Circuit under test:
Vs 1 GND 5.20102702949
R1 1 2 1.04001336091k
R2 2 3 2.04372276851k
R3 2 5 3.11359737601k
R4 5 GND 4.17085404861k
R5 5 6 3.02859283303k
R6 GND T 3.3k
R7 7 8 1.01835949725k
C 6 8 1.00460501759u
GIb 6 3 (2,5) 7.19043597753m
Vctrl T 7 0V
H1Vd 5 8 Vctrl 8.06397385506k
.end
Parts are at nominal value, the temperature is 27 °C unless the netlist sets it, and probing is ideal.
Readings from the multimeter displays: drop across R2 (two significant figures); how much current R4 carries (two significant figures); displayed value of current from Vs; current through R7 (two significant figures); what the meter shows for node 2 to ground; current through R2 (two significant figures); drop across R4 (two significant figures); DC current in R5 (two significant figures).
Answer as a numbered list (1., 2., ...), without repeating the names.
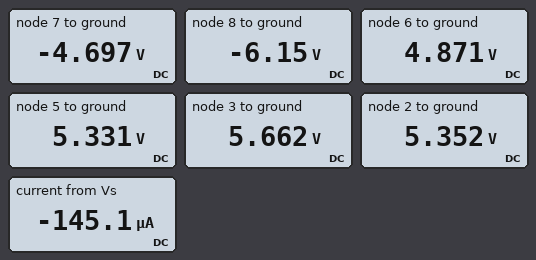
1. 310 mV
2. 1.3 mA
3. -145.1 µA
4. 1.4 mA
5. 5.352 V
6. 150 µA
7. 5.3 V
8. 150 µA
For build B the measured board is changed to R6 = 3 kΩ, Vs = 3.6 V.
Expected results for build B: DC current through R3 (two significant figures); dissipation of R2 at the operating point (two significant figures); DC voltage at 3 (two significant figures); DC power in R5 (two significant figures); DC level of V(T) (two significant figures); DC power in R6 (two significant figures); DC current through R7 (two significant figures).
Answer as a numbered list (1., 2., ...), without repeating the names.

1. 1.3 µA
2. 1.6 µW
3. 3.7 V
4. 2.4 µW
5. -2.7 V
6. 2.4 mW
7. 900 µA
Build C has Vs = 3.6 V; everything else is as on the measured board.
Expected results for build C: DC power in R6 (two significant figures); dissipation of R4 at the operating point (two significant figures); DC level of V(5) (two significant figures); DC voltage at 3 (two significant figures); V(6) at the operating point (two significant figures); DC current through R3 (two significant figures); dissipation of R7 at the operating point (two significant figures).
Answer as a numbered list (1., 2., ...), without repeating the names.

1. 3.2 mW
2. 3.3 mW
3. 3.7 V
4. 3.9 V
5. 3.4 V
6. 4.7 µA
7. 990 µW
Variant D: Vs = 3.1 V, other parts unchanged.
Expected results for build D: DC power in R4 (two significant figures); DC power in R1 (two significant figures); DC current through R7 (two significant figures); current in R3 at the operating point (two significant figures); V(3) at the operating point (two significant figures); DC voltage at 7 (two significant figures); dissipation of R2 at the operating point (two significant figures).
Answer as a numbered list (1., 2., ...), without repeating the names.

1. 2.4 mW
2. 7.8 µW
3. 850 µA
4. 4.0 µA
5. 3.4 V
6. -2.8 V
7. 17 µW
